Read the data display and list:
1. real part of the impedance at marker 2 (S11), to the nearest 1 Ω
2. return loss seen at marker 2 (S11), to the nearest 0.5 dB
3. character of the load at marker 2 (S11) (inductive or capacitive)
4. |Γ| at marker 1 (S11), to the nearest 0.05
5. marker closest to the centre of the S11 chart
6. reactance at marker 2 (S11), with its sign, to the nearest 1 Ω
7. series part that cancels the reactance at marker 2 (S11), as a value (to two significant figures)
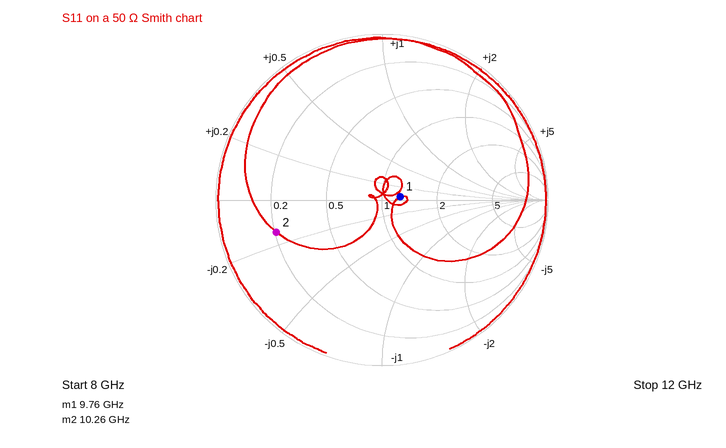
10 Ω
3.5 dB
capacitive
0.10
marker 1
-7 Ω
110 pH
